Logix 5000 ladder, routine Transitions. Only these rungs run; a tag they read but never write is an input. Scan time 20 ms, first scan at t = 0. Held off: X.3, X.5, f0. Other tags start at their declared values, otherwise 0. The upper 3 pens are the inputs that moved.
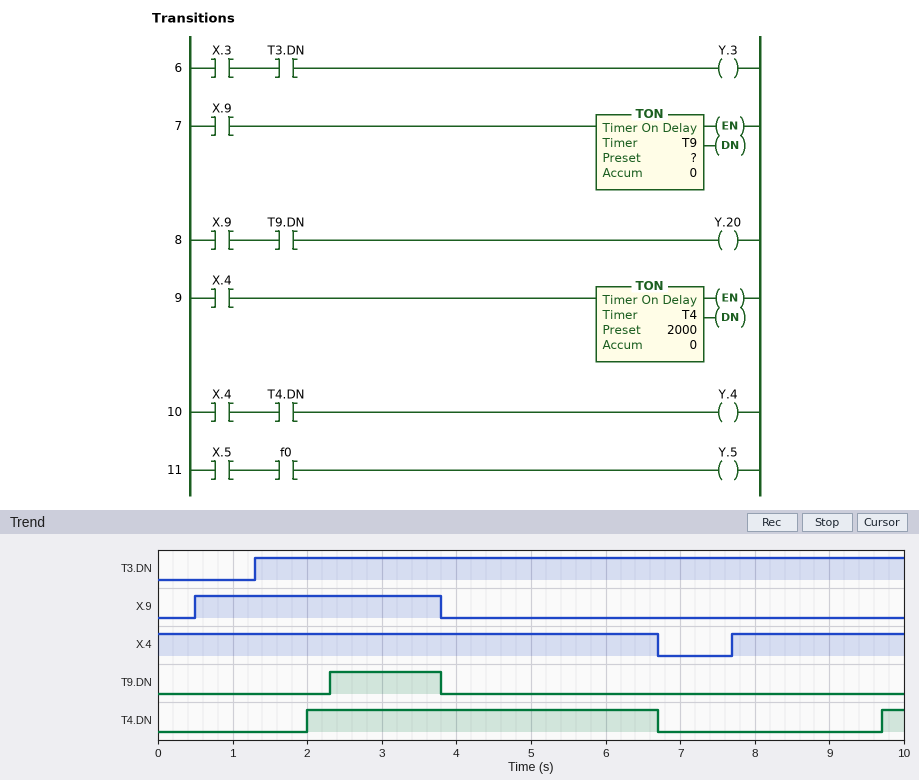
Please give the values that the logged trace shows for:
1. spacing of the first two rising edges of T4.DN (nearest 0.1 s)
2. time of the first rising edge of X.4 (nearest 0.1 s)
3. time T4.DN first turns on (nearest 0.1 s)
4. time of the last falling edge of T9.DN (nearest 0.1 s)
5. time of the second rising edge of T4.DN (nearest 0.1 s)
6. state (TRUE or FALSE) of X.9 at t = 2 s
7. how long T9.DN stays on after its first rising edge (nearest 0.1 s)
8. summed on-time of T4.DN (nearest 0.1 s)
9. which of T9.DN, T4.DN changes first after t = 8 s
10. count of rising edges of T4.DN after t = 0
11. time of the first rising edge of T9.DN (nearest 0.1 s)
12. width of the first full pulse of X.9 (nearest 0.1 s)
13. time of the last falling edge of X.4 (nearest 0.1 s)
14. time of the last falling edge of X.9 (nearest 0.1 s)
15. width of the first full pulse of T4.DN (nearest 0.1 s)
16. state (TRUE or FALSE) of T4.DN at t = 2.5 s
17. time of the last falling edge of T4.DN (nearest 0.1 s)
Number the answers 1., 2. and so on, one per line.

1. 7.7 s
2. 7.7 s
3. 2.0 s
4. 3.8 s
5. 9.7 s
6. TRUE
7. 1.5 s
8. 5.0 s
9. T4.DN
10. 2
11. 2.3 s
12. 3.3 s
13. 6.7 s
14. 3.8 s
15. 4.7 s
16. TRUE
17. 6.7 s
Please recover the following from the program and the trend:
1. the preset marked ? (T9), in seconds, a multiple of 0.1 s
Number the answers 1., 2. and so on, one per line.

1. 1.8 s
